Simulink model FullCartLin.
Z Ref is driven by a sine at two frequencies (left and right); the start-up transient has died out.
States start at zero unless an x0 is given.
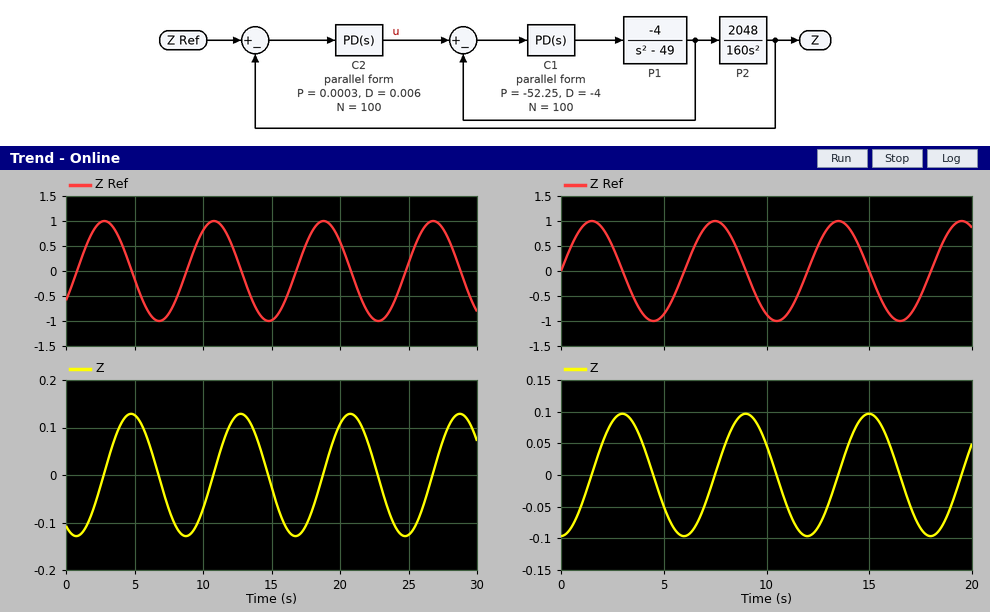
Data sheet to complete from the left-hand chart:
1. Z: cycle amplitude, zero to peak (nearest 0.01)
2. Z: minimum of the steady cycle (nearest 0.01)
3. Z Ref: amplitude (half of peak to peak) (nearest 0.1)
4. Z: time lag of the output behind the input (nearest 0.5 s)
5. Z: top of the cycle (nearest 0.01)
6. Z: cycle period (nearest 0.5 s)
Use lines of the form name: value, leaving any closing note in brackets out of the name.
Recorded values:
Z: cycle amplitude, zero to peak: 0.13
Z: minimum of the steady cycle: -0.13
Z Ref: amplitude (half of peak to peak): 1.0
Z: time lag of the output behind the input: 2.0 s
Z: top of the cycle: 0.13
Z: cycle period: 8.0 s
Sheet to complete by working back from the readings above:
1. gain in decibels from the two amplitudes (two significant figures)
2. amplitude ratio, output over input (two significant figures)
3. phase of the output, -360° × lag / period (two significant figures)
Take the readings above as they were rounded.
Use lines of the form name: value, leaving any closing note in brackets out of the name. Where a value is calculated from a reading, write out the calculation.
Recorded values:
gain in decibels from the two amplitudes: 20 log10(0.13 / 1) = -18 dB
amplitude ratio, output over input: 0.13 / 1 = 0.13
phase of the output, -360° × lag / period: -360 × 2 / 8 = -90°
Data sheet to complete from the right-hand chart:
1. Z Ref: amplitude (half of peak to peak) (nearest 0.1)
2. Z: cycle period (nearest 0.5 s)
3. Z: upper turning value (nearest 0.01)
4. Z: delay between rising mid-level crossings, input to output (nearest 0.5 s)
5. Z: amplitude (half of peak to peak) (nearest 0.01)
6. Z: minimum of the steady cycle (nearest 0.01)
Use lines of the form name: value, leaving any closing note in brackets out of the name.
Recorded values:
Z Ref: amplitude (half of peak to peak): 1.0
Z: cycle period: 6.0 s
Z: upper turning value: 0.10
Z: delay between rising mid-level crossings, input to output: 1.5 s
Z: amplitude (half of peak to peak): 0.10
Z: minimum of the steady cycle: -0.10
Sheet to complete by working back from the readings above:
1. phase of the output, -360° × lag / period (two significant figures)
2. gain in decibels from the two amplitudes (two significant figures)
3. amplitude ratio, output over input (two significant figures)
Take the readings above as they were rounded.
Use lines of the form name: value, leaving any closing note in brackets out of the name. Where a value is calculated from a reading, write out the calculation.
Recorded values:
phase of the output, -360° × lag / period: -360 × 1.5 / 6 = -90°
gain in decibels from the two amplitudes: 20 log10(0.1 / 1) = -20 dB
amplitude ratio, output over input: 0.1 / 1 = 0.10
